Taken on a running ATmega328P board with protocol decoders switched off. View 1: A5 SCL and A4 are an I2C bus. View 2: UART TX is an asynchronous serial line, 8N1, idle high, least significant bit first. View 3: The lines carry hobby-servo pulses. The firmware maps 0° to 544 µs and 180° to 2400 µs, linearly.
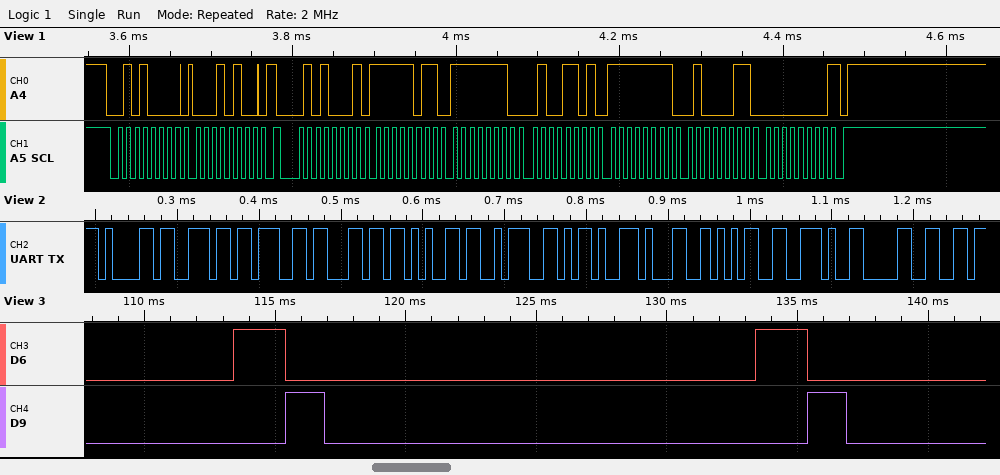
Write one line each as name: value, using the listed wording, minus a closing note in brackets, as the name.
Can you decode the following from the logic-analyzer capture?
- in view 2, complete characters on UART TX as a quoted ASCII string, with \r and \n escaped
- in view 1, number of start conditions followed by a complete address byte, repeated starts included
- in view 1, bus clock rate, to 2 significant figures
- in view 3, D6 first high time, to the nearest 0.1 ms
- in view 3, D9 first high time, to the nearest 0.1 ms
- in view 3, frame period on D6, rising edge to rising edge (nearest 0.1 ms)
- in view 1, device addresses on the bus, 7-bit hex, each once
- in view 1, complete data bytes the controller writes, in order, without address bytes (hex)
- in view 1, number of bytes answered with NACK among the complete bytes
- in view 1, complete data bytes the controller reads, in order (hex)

in view 2, complete characters on UART TX as a quoted ASCII string, with \r and \n escaped: "angle:-15.0"
in view 1, number of start conditions followed by a complete address byte, repeated starts included: 2
in view 1, bus clock rate, to 2 significant figures: 100 kHz
in view 3, D6 first high time, to the nearest 0.1 ms: 2.0 ms
in view 3, D9 first high time, to the nearest 0.1 ms: 1.5 ms
in view 3, frame period on D6, rising edge to rising edge: 20.0 ms
in view 1, device addresses on the bus, 7-bit hex, each once: 0x28
in view 1, complete data bytes the controller writes, in order, without address bytes: 14
in view 1, number of bytes answered with NACK among the complete bytes: 1
in view 1, complete data bytes the controller reads, in order: FB FE 4D FF 43 00
